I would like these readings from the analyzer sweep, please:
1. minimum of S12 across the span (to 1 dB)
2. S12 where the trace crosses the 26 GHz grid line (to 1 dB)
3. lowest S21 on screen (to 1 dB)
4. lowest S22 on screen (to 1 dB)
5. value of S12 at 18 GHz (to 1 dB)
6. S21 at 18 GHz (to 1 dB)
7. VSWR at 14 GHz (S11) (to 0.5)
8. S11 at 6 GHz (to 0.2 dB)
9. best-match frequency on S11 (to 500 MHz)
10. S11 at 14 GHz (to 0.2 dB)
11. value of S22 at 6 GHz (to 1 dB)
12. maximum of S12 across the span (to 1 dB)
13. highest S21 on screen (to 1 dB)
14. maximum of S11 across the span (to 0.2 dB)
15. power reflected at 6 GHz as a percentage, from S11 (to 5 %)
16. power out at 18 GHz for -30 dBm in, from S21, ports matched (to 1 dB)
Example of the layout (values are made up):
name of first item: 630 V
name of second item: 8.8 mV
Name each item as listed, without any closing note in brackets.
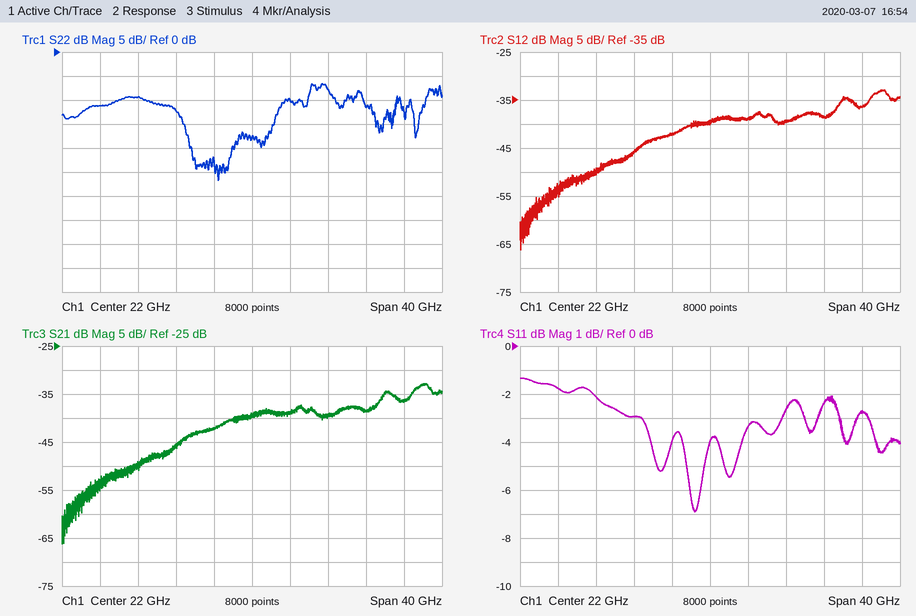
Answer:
minimum of S12 across the span: -66 dB
S12 where the trace crosses the 26 GHz grid line: -39 dB
lowest S21 on screen: -66 dB
lowest S22 on screen: -27 dB
value of S12 at 18 GHz: -42 dB
S21 at 18 GHz: -42 dB
VSWR at 14 GHz (S11): 6.0
S11 at 6 GHz: -1.8 dB
best-match frequency on S11: 20.5 GHz
S11 at 14 GHz: -3.0 dB
value of S22 at 6 GHz: -11 dB
maximum of S12 across the span: -33 dB
highest S21 on screen: -33 dB
maximum of S11 across the span: -1.4 dB
power reflected at 6 GHz as a percentage, from S11: 65 %
power out at 18 GHz for -30 dBm in, from S21, ports matched: -72 dBm
